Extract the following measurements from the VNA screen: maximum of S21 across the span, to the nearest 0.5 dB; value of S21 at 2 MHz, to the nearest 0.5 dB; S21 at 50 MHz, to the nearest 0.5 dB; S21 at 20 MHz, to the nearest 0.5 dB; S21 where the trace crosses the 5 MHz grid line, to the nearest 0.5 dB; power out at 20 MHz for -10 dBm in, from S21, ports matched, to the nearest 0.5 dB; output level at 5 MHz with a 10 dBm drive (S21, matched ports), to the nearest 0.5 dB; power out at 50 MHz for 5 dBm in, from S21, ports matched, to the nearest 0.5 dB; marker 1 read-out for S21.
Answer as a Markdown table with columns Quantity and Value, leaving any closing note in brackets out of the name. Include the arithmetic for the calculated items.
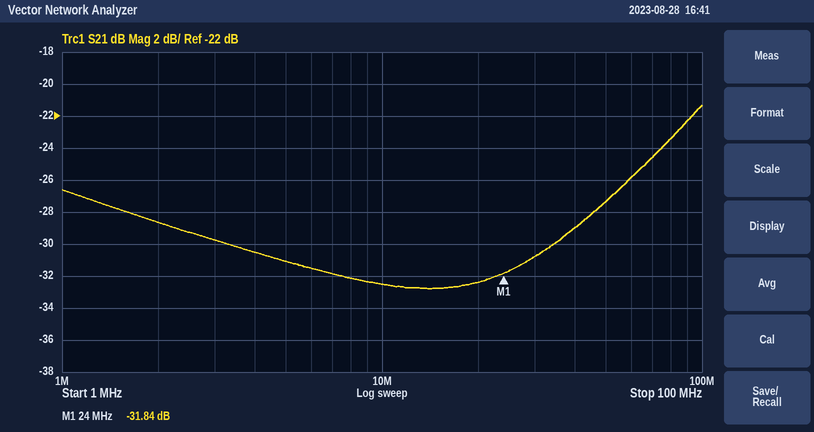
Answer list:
| Quantity | Value |
|---|---|
| maximum of S21 across the span, to the nearest 0.5 dB | -21.5 dB |
| value of S21 at 2 MHz, to the nearest 0.5 dB | -28.5 dB |
| S21 at 50 MHz, to the nearest 0.5 dB | -27.5 dB |
| S21 at 20 MHz, to the nearest 0.5 dB | -32.5 dB |
| S21 where the trace crosses the 5 MHz grid line, to the nearest 0.5 dB | -31.0 dB |
| power out at 20 MHz for -10 dBm in, from S21, ports matched, to the nearest 0.5 dB | -10 dBm + (-32.5 dB) = -42.5 dBm |
| output level at 5 MHz with a 10 dBm drive (S21, matched ports), to the nearest 0.5 dB | 10 dBm + (-31.0 dB) = -21.0 dBm |
| power out at 50 MHz for 5 dBm in, from S21, ports matched, to the nearest 0.5 dB | 5 dBm + (-27.5 dB) = -22.5 dBm |
| marker 1 read-out for S21 | -31.84 dB |
